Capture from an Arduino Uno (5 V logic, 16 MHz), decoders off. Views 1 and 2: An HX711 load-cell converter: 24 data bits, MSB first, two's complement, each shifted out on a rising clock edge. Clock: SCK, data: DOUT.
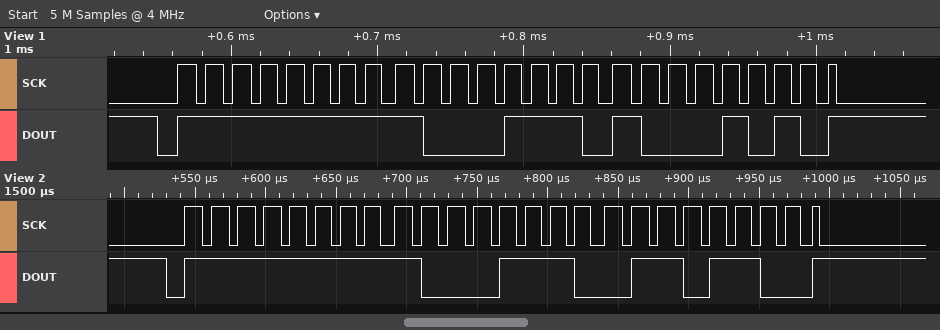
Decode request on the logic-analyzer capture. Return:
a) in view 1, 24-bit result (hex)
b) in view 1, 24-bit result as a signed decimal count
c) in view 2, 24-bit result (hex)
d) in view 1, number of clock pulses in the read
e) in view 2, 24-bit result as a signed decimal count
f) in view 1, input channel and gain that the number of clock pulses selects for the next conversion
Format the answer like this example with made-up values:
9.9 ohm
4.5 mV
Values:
0xFF8E8A
-29046
0xFF8E6C
25
-29076
channel A, gain 128
